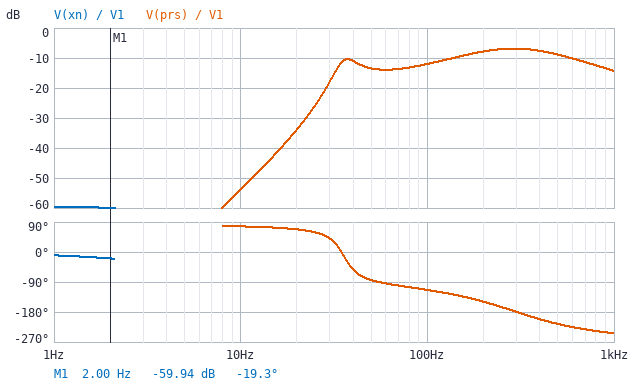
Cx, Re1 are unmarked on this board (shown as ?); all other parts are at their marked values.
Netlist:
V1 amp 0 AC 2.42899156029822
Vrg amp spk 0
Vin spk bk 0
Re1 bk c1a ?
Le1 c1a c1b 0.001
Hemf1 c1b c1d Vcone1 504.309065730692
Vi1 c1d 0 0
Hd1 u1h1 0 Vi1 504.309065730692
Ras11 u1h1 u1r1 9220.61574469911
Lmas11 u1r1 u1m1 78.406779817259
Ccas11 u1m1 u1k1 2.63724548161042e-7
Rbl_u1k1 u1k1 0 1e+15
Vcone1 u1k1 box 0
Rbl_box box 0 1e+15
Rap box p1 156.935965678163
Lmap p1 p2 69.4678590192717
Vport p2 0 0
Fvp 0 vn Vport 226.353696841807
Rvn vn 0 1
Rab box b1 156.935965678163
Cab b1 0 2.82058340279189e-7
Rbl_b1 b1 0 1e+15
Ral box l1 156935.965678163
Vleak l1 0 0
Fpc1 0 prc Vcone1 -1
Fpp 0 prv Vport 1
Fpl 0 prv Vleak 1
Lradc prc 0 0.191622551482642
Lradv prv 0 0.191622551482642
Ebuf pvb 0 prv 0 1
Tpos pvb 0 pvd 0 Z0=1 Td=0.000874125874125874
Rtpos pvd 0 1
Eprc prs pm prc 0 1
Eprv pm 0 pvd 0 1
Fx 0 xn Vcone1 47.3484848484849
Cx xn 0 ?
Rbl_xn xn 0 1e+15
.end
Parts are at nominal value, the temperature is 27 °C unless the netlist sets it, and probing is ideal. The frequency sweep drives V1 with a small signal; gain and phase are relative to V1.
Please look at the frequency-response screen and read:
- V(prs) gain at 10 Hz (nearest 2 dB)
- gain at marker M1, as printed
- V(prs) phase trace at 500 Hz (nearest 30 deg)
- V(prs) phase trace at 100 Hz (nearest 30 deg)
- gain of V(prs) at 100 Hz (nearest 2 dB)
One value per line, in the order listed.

-54 dB
-59.94 dB
-210 deg
-120 deg
-12 dB
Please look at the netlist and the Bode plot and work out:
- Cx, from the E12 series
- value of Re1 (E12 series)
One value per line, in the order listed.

2.2 F
2.7 Ω
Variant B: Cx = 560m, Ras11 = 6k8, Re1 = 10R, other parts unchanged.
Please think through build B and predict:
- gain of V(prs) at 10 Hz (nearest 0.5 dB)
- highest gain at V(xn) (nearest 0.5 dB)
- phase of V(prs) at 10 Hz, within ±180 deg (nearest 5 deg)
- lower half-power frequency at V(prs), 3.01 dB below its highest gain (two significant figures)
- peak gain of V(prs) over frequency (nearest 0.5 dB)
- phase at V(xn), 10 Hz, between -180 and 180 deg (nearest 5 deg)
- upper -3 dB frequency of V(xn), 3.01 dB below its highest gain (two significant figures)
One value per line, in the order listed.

-59.5 dB
-59.0 dB
110 deg
37 Hz
-15.5 dB
-35 deg
24 Hz
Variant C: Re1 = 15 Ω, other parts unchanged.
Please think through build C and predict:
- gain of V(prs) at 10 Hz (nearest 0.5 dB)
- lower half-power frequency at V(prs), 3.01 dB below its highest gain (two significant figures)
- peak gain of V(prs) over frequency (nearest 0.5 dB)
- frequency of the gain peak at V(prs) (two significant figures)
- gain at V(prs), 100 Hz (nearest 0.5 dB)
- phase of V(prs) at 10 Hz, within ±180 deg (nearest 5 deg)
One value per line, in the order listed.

-62.5 dB
40 Hz
-17.5 dB
56 Hz
-19.5 dB
115 deg
